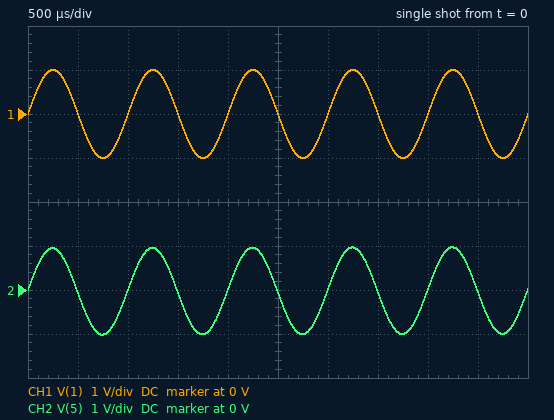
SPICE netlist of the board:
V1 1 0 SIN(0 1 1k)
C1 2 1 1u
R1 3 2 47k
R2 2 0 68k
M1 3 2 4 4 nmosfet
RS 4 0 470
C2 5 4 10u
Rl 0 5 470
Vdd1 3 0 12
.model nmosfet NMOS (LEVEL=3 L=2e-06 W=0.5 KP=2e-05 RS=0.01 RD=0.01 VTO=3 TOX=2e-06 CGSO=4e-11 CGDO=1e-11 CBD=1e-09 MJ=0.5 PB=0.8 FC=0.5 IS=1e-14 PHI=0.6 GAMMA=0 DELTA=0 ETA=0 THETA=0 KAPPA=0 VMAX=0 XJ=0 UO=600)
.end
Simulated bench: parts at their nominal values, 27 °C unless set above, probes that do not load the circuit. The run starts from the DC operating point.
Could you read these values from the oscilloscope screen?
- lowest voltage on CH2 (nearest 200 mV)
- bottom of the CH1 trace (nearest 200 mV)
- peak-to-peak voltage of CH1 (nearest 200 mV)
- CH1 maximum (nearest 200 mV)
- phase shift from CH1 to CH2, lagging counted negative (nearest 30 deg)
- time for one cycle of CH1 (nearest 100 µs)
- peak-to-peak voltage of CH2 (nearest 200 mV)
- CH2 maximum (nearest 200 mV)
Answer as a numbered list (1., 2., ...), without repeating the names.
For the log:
1. -1.0 V
2. -1.0 V
3. 2.0 V
4. 1.0 V
5. 0 deg
6. 1.0 ms
7. 2.0 V
8. 1.0 V
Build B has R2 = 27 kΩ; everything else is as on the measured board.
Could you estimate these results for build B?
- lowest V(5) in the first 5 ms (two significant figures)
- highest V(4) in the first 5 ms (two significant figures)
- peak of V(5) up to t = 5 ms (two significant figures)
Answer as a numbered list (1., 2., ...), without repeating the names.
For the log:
1. -700 mV
2. 2.3 V
3. 940 mV
